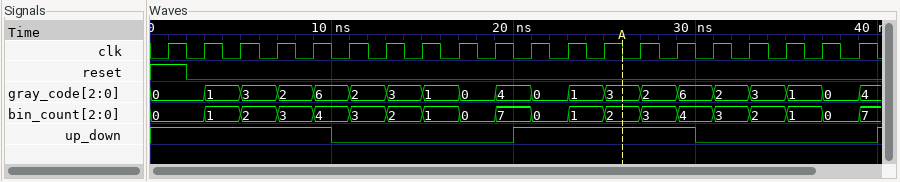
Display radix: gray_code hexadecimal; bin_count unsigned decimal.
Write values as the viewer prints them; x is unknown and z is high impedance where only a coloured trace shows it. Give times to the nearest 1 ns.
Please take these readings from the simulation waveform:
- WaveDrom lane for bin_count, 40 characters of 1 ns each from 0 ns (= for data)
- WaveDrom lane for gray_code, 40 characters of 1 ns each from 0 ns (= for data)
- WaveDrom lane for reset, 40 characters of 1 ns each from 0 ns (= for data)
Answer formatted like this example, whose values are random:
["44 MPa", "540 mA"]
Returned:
["{name: 'bin_count', wave: '=..=.=.=.=.=.=.=.=.=.=.=.=.=.=.=.=.=.=.=', data: '0 1 2 3 4 3 2 1 0 7 0 1 2 3 4 3 2 1 0 7'}", "{name: 'gray_code', wave: '=..=.=.=.=.=.=.=.=.=.=.=.=.=.=.=.=.=.=.=', data: '0 1 3 2 6 2 3 1 0 4 0 1 3 2 6 2 3 1 0 4'}", "{name: 'reset', wave: '1.0.....................................'}"]
